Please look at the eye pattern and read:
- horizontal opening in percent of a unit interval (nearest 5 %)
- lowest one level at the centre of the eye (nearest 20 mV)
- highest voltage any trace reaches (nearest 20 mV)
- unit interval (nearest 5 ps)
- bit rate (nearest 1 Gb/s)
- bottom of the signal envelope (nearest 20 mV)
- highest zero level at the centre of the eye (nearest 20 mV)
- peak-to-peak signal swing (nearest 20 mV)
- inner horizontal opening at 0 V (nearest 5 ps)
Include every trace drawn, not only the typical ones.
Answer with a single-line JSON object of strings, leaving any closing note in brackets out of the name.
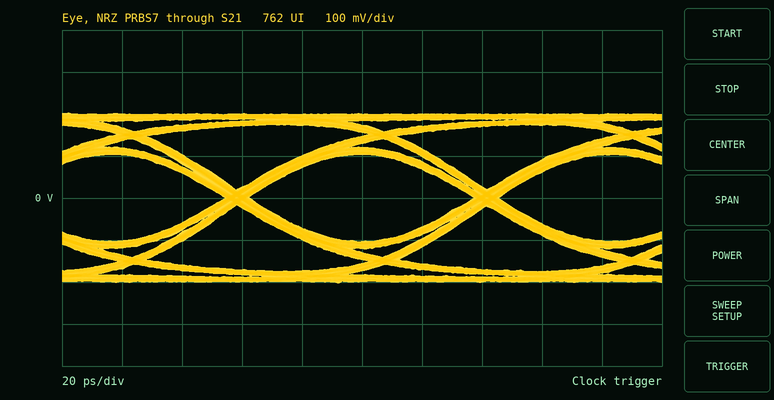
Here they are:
{"horizontal opening in percent of a unit interval": "90 %", "lowest one level at the centre of the eye": "100 mV", "highest voltage any trace reaches": "200 mV", "unit interval": "85 ps", "bit rate": "12 Gb/s", "bottom of the signal envelope": "-200 mV", "highest zero level at the centre of the eye": "-100 mV", "peak-to-peak signal swing": "400 mV", "inner horizontal opening at 0 V": "75 ps"}
